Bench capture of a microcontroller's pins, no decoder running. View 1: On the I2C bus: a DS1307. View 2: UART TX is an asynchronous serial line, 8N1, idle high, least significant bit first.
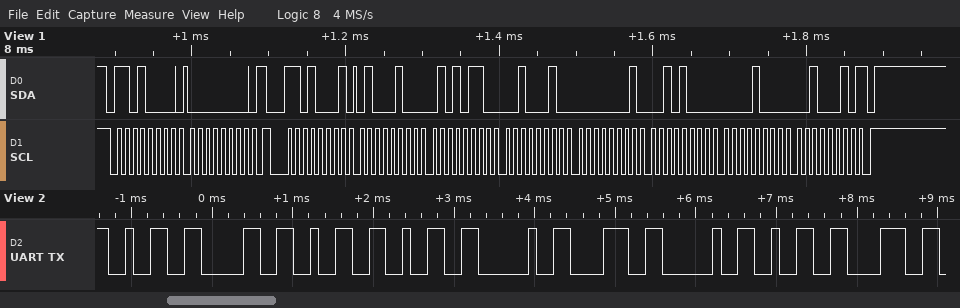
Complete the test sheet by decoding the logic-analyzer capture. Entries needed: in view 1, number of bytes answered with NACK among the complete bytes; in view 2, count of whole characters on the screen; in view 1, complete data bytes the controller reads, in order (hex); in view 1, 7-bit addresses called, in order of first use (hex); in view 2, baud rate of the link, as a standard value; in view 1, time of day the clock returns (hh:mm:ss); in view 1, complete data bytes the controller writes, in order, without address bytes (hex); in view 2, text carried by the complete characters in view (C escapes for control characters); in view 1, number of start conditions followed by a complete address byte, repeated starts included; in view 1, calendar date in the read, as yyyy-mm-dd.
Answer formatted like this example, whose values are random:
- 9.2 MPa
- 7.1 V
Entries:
- 1
- 9
- 44 56 22 01 28 08 22
- 0x68
- 9600 baud
- 22:56:44
- 00
- "2022 8 28"
- 2
- 2022-08-28
